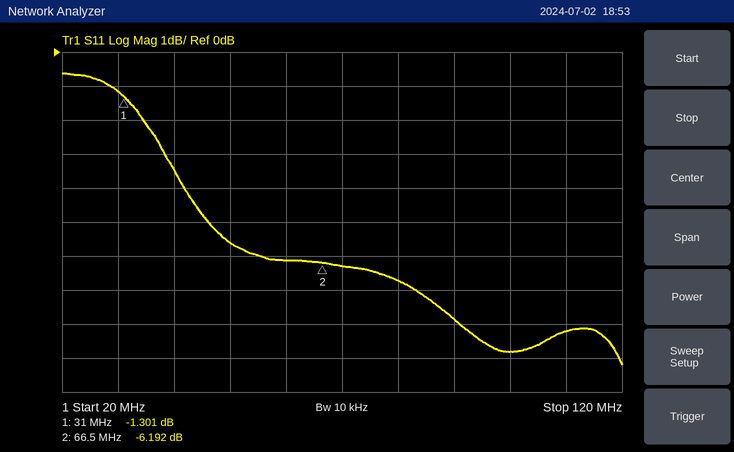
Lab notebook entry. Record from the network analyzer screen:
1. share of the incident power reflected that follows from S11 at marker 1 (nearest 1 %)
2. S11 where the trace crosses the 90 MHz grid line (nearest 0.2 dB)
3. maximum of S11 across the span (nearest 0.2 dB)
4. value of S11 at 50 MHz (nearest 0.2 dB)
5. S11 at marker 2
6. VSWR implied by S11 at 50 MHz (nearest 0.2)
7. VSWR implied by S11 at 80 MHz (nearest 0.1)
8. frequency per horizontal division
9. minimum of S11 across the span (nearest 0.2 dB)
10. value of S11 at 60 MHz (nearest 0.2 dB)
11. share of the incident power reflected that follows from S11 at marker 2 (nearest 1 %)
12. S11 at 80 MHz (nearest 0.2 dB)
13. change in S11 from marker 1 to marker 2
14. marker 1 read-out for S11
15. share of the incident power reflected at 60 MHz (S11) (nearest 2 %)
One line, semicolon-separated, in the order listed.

74 %; -7.8 dB; -0.6 dB; -5.6 dB; -6.192 dB; 3.2; 2.7; 10 MHz; -9.2 dB; -6.2 dB; 24 %; -6.8 dB; -4.891 dB; -1.301 dB; 24 %
